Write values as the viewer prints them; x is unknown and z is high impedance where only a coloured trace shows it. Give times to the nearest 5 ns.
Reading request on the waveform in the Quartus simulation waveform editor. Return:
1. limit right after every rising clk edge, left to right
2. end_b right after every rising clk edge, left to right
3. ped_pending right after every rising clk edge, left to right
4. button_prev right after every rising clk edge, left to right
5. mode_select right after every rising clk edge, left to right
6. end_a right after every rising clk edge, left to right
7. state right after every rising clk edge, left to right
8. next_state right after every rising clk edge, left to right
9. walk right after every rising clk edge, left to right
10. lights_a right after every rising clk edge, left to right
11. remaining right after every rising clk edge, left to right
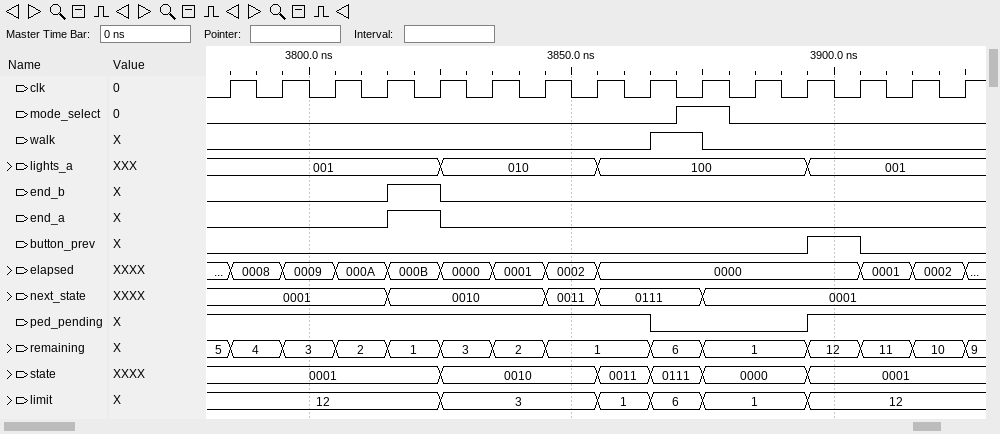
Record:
12, 12, 12, 12, 3, 3, 3, 1, 6, 1, 1, 12, 12, 12, 12
0 0 0 1 0 0 0 0 0 0 0 0 0 0 0
1 1 1 1 1 1 1 1 0 0 0 1 1 1 1
0 0 0 0 0 0 0 0 0 0 0 1 0 0 0
0 0 0 0 0 0 0 0 0 1 0 0 0 0 0
0 0 0 1 0 0 0 0 0 0 0 0 0 0 0
0001, 0001, 0001, 0001, 0010, 0010, 0010, 0011, 0111, 0000, 0000, 0001, 0001, 0001, 0001
0001, 0001, 0001, 0010, 0010, 0010, 0011, 0111, 0111, 0001, 0001, 0001, 0001, 0001, 0001
0 0 0 0 0 0 0 0 1 0 0 0 0 0 0
001, 001, 001, 001, 010, 010, 010, 100, 100, 100, 100, 001, 001, 001, 001
4, 3, 2, 1, 3, 2, 1, 1, 6, 1, 1, 12, 11, 10, 9
